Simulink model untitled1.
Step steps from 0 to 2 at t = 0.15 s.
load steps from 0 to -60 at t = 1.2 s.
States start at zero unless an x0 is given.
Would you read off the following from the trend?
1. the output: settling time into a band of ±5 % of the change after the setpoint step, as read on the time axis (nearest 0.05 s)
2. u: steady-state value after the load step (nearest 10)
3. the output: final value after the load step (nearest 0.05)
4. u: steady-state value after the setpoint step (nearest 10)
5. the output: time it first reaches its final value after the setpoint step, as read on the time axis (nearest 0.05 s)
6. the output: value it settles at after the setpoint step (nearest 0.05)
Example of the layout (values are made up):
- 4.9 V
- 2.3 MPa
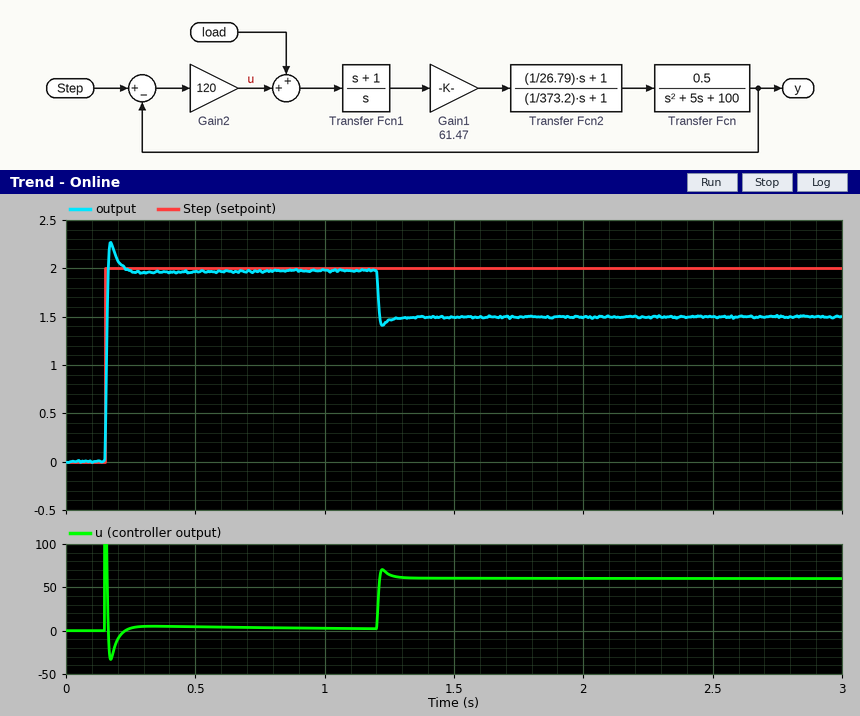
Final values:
- 0.20 s
- 60
- 1.50
- 0
- 0.15 s
- 2.00
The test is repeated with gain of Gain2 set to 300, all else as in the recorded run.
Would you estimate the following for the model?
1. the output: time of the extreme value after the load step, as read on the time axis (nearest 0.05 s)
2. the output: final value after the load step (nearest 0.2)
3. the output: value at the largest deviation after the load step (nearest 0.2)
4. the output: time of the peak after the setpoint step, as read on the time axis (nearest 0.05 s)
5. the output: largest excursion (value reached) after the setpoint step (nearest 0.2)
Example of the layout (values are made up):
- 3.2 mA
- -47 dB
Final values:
- 1.20 s
- 1.8
- 1.8
- 0.15 s
- 2.4
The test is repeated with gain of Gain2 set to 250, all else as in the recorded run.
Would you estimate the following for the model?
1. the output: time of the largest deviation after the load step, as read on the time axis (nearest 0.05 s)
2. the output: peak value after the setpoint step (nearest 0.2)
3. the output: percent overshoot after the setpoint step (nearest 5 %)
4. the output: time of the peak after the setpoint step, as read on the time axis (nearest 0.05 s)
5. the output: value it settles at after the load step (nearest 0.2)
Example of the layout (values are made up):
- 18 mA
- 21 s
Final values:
- 1.20 s
- 2.4
- 20 %
- 0.15 s
- 1.8
